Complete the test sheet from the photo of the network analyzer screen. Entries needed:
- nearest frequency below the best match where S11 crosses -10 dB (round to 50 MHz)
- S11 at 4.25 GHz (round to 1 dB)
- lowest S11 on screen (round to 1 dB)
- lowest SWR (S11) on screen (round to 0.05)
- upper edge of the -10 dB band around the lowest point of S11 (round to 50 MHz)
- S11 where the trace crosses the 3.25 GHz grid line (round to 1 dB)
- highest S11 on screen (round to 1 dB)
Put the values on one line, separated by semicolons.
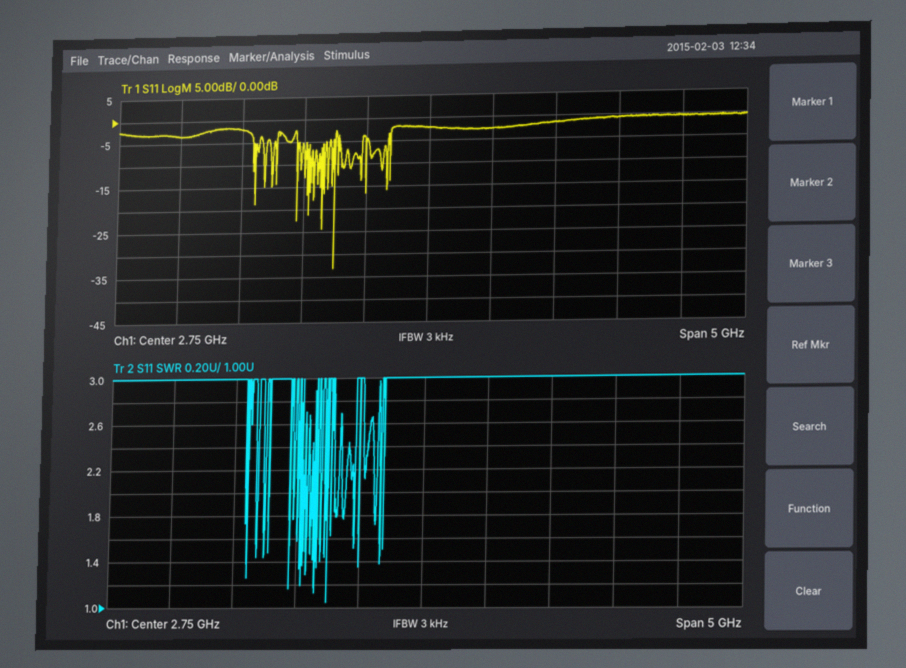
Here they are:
2.00 GHz; -1 dB; -33 dB; 1.05; 2.00 GHz; -3 dB; 0 dB
